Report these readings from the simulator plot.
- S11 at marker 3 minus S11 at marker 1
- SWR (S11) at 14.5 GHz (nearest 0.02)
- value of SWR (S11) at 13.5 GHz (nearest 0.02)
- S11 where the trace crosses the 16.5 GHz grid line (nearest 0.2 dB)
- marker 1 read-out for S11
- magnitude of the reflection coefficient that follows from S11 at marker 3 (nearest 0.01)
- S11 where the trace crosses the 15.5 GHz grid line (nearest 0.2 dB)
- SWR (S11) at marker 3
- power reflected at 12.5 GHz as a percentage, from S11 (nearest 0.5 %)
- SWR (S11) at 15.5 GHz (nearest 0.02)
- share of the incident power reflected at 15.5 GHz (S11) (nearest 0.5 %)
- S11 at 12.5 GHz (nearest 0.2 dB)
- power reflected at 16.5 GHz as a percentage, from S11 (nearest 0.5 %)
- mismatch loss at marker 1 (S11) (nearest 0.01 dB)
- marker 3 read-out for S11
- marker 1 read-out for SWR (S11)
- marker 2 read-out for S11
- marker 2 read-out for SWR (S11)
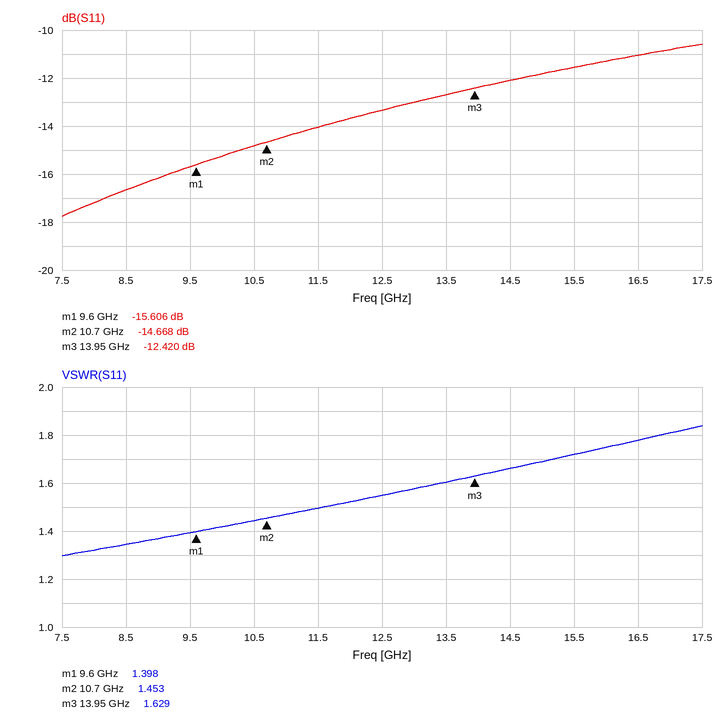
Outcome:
3.186 dB
1.66
1.60
-11.0 dB
-15.606 dB
0.24
-11.6 dB
1.629
4.5 %
1.72
7.0 %
-13.4 dB
8.0 %
0.12 dB
-12.420 dB
1.398
-14.668 dB
1.453
